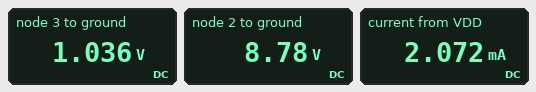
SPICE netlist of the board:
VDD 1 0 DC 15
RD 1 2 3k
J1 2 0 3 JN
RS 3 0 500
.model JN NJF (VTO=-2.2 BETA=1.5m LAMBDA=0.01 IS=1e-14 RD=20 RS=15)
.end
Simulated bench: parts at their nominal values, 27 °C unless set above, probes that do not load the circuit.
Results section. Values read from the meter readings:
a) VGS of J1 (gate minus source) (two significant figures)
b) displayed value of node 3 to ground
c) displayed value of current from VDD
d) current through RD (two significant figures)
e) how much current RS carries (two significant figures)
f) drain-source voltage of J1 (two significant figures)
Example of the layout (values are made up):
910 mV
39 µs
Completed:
-1.0 V
1.036 V
2.072 mA
2.1 mA
2.1 mA
7.7 V
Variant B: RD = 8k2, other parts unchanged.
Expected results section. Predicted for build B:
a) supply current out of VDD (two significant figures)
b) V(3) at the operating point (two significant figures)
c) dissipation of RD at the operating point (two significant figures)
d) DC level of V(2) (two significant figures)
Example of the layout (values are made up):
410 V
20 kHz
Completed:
1.7 mA
830 mV
23 mW
1.4 V
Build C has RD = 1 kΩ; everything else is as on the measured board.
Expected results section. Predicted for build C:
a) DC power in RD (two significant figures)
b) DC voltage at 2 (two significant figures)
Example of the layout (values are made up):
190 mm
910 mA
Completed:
4.4 mW
13 V
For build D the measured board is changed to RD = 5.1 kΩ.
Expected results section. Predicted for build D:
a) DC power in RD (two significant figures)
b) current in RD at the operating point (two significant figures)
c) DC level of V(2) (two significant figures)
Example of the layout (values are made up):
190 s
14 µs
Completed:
21 mW
2.0 mA
4.6 V
